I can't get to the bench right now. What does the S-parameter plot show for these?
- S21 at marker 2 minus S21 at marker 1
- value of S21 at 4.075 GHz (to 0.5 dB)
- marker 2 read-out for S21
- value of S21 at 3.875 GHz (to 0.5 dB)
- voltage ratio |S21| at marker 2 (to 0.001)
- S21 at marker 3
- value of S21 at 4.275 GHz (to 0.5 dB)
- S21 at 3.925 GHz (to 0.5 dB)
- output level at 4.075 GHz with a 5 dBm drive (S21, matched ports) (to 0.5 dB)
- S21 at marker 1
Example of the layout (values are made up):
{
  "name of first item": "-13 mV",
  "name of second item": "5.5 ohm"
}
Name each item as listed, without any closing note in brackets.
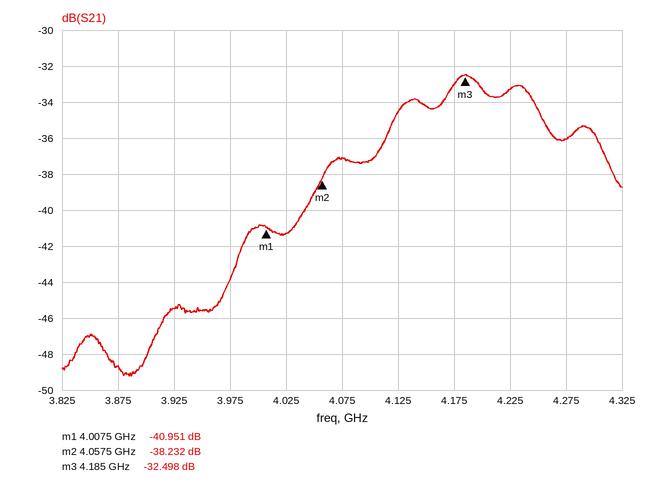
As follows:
{
  "S21 at marker 2 minus S21 at marker 1": "2.719 dB",
  "value of S21 at 4.075 GHz": "-37.0 dB",
  "marker 2 read-out for S21": "-38.232 dB",
  "value of S21 at 3.875 GHz": "-48.5 dB",
  "voltage ratio |S21| at marker 2": "0.012",
  "S21 at marker 3": "-32.498 dB",
  "value of S21 at 4.275 GHz": "-36.0 dB",
  "S21 at 3.925 GHz": "-45.5 dB",
  "output level at 4.075 GHz with a 5 dBm drive (S21, matched ports)": "-32.0 dBm",
  "S21 at marker 1": "-40.951 dB"
}
